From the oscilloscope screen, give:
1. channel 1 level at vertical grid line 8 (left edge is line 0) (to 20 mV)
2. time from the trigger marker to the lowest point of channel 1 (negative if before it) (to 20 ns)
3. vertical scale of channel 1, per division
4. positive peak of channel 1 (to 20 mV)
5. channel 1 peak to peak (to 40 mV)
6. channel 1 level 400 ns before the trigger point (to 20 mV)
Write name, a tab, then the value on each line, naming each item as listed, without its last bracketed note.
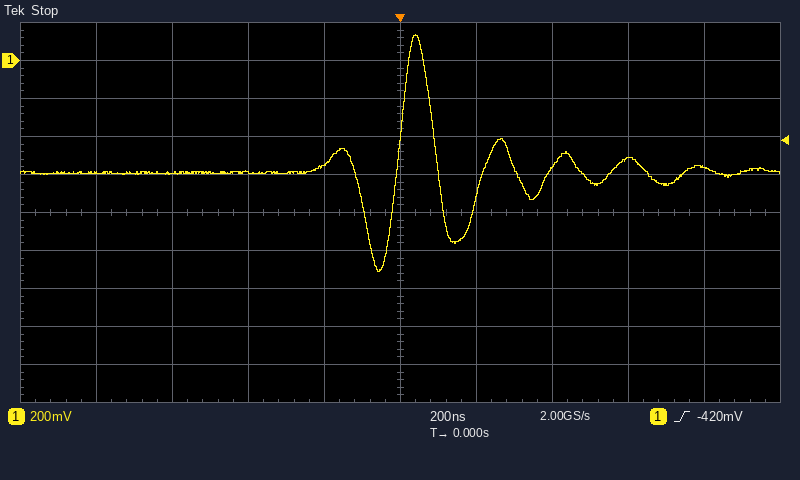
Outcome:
channel 1 level at vertical grid line 8 (left edge is line 0)	-520 mV
time from the trigger marker to the lowest point of channel 1 (negative if before it)	-60 ns
vertical scale of channel 1, per division	200 mV
positive peak of channel 1	140 mV
channel 1 peak to peak	1.24 V
channel 1 level 400 ns before the trigger point	-580 mV
